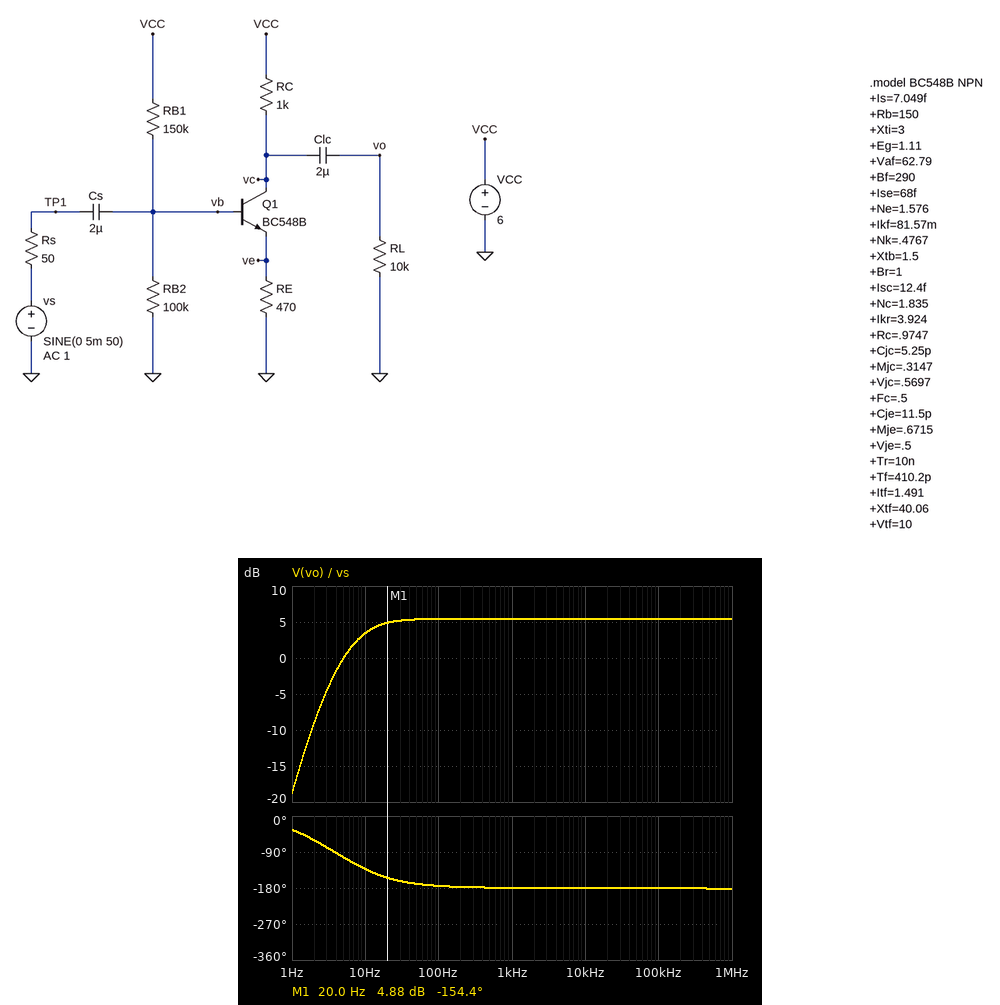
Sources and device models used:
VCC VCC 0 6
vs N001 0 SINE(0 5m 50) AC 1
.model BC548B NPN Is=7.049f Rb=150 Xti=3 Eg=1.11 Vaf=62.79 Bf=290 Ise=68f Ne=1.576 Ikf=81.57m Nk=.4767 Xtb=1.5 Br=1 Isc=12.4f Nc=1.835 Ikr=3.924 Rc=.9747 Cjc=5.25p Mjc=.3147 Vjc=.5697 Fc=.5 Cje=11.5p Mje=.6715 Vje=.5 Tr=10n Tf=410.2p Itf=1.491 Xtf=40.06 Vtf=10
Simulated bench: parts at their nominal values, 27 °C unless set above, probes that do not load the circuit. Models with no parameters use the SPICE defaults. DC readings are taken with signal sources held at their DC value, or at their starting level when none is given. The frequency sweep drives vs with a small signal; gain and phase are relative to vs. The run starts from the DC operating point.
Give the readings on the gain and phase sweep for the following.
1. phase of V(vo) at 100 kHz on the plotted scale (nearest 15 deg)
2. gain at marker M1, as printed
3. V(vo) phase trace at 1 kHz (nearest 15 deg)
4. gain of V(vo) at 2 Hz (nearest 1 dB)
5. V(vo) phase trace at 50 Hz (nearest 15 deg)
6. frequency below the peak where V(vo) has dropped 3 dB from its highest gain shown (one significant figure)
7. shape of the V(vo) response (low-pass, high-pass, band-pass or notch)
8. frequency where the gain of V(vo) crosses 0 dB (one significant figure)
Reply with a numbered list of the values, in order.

1. -180 deg
2. 4.88 dB
3. -180 deg
4. -9 dB
5. -165 deg
6. 8 Hz
7. high-pass
8. 5 Hz
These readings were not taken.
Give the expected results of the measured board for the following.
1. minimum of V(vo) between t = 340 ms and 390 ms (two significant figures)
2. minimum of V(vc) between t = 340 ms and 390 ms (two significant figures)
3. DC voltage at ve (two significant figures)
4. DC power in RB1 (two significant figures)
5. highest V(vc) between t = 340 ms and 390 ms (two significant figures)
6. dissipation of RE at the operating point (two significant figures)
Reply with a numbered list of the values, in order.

1. -9.3 mV
2. 3.6 V
3. 1.1 V
4. 120 µW
5. 3.6 V
6. 2.7 mW
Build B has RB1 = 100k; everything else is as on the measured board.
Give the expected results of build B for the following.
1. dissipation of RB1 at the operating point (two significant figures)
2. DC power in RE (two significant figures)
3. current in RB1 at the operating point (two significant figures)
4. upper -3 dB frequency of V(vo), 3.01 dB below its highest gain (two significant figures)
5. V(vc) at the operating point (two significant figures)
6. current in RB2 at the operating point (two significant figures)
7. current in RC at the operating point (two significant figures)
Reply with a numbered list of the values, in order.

1. 140 µW
2. 5.5 mW
3. 37 µA
4. 26 MHz
5. 2.6 V
6. 23 µA
7. 3.4 mA
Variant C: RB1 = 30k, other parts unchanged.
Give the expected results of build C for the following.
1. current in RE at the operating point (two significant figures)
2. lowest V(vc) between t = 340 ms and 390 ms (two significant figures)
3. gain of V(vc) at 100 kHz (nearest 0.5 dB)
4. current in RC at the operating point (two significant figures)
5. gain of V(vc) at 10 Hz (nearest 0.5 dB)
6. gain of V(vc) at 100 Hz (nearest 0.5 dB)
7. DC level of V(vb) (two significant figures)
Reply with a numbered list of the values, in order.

1. 4.1 mA
2. 2.0 V
3. -19.0 dB
4. 4.0 mA
5. -41.0 dB
6. -23.0 dB
7. 2.6 V
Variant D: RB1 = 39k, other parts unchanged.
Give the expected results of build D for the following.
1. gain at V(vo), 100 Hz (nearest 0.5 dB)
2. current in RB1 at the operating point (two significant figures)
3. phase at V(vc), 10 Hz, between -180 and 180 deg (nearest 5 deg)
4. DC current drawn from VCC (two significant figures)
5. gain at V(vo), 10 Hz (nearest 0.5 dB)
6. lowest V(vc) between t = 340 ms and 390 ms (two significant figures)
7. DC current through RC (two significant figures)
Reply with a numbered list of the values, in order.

1. -24.5 dB
2. 87 µA
3. -95 deg
4. 4.1 mA
5. -44.0 dB
6. 2.0 V
7. 4.0 mA
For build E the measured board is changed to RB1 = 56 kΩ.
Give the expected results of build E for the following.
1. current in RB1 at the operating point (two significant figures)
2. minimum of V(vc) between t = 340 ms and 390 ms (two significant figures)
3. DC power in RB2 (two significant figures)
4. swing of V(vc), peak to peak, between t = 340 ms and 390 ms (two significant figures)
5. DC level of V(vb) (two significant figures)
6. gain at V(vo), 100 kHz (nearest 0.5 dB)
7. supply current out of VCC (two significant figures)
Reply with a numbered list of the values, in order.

1. 61 µA
2. 2.0 V
3. 67 µW
4. 3.1 mV
5. 2.6 V
6. -4.5 dB
7. 4.0 mA
